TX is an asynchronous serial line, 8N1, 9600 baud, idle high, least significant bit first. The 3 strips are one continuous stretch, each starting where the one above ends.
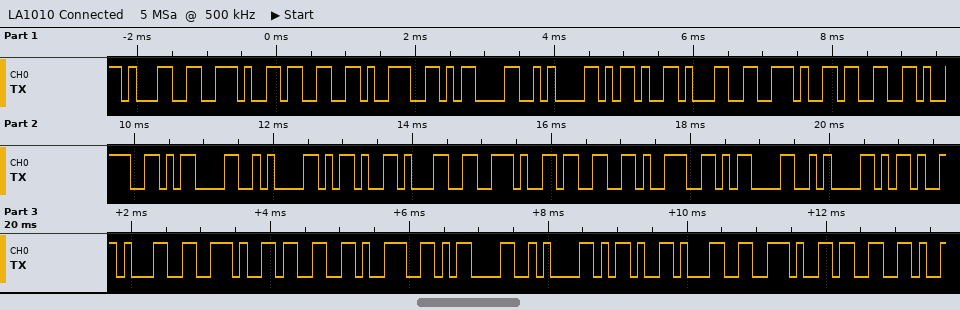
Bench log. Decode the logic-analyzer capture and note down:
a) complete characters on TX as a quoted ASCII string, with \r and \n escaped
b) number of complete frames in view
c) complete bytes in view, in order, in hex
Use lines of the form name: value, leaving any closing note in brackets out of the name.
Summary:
complete characters on TX as a quoted ASCII string, with \r and \n escaped: "1.39\r\n-1.39\r\n-1.39\r\n-1.39\r\n-1.3"
number of complete frames in view: 31
complete bytes in view, in order, in hex: 0x31 0x2E 0x33 0x39 0x0D 0x0A 0x2D 0x31 0x2E 0x33 0x39 0x0D 0x0A 0x2D 0x31 0x2E 0x33 0x39 0x0D 0x0A 0x2D 0x31 0x2E 0x33 0x39 0x0D 0x0A 0x2D 0x31 0x2E 0x33
